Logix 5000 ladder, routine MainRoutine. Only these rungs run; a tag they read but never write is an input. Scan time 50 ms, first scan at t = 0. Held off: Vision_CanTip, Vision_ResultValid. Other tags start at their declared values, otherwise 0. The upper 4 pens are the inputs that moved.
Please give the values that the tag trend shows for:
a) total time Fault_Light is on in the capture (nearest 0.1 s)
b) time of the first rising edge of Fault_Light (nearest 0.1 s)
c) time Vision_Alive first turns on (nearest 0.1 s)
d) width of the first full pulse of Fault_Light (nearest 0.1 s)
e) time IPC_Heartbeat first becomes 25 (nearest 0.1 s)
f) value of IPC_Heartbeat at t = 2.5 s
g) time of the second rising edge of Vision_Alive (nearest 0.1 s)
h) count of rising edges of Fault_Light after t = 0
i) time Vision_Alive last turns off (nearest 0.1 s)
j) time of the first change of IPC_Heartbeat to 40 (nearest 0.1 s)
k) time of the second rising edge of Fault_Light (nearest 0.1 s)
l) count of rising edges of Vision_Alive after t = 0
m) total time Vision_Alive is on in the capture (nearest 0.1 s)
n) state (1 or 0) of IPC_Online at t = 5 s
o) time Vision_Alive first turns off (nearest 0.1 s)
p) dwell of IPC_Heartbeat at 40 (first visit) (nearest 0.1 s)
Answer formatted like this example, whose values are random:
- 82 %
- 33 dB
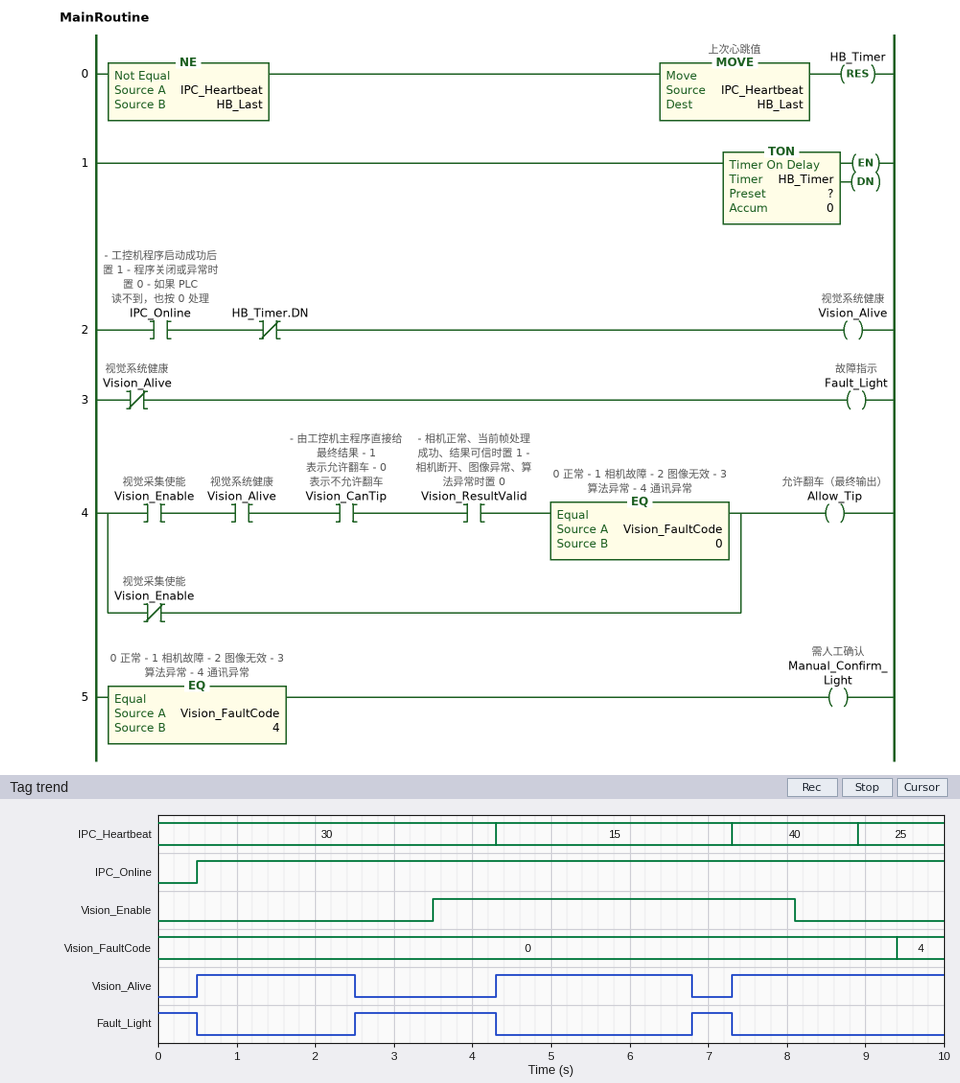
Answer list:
- 2.8 s
- 2.5 s
- 0.5 s
- 1.8 s
- 8.9 s
- 30
- 4.3 s
- 2
- 6.8 s
- 7.3 s
- 6.8 s
- 3
- 7.2 s
- 1
- 2.5 s
- 1.6 s
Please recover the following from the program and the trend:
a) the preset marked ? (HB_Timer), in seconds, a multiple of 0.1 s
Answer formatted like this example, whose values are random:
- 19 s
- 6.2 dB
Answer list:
- 2.5 s
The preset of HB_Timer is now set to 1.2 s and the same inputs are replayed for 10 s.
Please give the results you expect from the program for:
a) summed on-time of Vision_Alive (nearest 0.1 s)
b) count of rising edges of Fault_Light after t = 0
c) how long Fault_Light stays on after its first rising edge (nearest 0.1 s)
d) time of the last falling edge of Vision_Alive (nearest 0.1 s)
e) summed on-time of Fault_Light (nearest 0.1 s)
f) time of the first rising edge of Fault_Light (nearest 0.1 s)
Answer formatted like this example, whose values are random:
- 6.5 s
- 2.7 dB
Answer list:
- 4.2 s
- 3
- 3.1 s
- 8.5 s
- 5.8 s
- 1.2 s
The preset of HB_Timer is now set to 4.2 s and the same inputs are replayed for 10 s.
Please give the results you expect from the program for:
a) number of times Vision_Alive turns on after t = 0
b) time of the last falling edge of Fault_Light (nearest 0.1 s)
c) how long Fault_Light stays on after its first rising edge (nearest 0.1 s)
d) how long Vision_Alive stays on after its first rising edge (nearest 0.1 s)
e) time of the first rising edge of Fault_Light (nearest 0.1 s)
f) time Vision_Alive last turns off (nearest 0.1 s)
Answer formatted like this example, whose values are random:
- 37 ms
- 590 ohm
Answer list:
- 2
- 4.3 s
- 0.1 s
- 3.7 s
- 4.2 s
- 4.2 s
